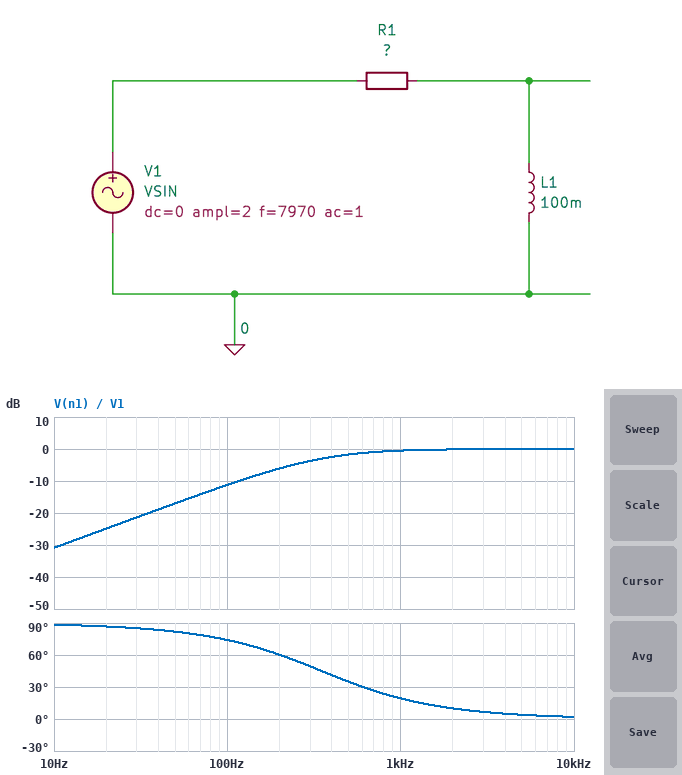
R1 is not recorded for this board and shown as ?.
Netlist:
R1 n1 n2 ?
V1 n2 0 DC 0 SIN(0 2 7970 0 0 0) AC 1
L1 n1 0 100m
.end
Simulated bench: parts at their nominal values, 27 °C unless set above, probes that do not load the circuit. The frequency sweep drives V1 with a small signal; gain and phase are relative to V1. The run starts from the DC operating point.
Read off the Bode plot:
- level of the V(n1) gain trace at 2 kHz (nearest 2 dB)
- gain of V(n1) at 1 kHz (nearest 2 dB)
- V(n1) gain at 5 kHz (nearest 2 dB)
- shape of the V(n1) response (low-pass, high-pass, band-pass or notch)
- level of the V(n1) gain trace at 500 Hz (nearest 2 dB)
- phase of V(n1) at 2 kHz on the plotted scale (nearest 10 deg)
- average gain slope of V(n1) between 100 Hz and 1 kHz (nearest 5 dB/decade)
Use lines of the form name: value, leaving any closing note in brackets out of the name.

level of the V(n1) gain trace at 2 kHz: 0 dB
gain of V(n1) at 1 kHz: 0 dB
V(n1) gain at 5 kHz: 0 dB
shape of the V(n1) response: high-pass
level of the V(n1) gain trace at 500 Hz: -2 dB
phase of V(n1) at 2 kHz on the plotted scale: 10 deg
average gain slope of V(n1) between 100 Hz and 1 kHz: 10 dB/decade
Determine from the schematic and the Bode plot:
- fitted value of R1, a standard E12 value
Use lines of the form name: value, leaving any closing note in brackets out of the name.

fitted value of R1, a standard E12 value: 220 Ω
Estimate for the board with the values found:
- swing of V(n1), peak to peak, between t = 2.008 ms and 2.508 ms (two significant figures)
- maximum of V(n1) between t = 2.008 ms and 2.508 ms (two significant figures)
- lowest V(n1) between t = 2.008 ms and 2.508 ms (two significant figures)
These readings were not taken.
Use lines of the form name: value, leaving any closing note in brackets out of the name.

swing of V(n1), peak to peak, between t = 2.008 ms and 2.508 ms: 4.0 V
maximum of V(n1) between t = 2.008 ms and 2.508 ms: 2.0 V
lowest V(n1) between t = 2.008 ms and 2.508 ms: -2.0 V
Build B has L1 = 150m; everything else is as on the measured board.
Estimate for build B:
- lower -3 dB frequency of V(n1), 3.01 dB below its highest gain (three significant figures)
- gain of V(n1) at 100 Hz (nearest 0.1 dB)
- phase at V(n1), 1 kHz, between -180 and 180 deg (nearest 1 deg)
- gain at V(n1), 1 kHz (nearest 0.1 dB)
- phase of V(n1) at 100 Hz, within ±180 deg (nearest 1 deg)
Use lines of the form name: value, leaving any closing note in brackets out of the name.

lower -3 dB frequency of V(n1), 3.01 dB below its highest gain: 233 Hz
gain of V(n1) at 100 Hz: -8.1 dB
phase at V(n1), 1 kHz, between -180 and 180 deg: 13 deg
gain at V(n1), 1 kHz: -0.2 dB
phase of V(n1) at 100 Hz, within ±180 deg: 67 deg
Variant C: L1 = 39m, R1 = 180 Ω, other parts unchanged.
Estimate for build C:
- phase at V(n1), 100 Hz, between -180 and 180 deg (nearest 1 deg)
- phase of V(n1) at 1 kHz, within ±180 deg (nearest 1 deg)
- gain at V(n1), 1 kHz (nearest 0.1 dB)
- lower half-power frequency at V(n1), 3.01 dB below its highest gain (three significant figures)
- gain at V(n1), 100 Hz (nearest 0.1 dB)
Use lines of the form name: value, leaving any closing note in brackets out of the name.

phase at V(n1), 100 Hz, between -180 and 180 deg: 82 deg
phase of V(n1) at 1 kHz, within ±180 deg: 36 deg
gain at V(n1), 1 kHz: -1.9 dB
lower half-power frequency at V(n1), 3.01 dB below its highest gain: 735 Hz
gain at V(n1), 100 Hz: -17.4 dB
